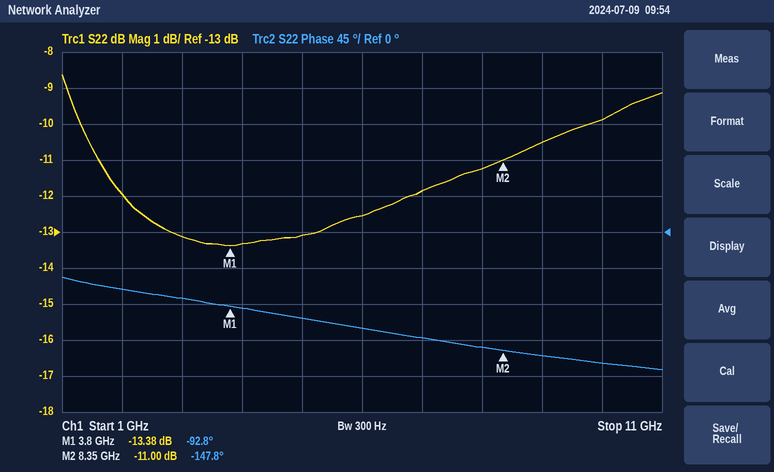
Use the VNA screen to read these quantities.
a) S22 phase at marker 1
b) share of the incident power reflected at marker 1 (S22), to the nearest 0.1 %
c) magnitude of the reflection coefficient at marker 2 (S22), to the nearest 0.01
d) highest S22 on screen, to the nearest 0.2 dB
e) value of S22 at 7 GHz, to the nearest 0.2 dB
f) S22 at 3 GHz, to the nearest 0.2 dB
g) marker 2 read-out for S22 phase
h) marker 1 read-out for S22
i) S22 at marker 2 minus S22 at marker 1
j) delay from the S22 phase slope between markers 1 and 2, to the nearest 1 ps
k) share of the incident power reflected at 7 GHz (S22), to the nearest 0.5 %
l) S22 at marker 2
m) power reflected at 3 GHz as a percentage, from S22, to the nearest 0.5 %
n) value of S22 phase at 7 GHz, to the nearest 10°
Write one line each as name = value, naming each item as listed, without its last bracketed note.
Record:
S22 phase at marker 1 = -92.8°
share of the incident power reflected at marker 1 (S22), to the nearest 0.1 % = 4.6 %
magnitude of the reflection coefficient at marker 2 (S22), to the nearest 0.01 = 0.28
highest S22 on screen, to the nearest 0.2 dB = -8.6 dB
value of S22 at 7 GHz, to the nearest 0.2 dB = -11.8 dB
S22 at 3 GHz, to the nearest 0.2 dB = -13.2 dB
marker 2 read-out for S22 phase = -147.8°
marker 1 read-out for S22 = -13.38 dB
S22 at marker 2 minus S22 at marker 1 = 2.38 dB
delay from the S22 phase slope between markers 1 and 2, to the nearest 1 ps = 34 ps
share of the incident power reflected at 7 GHz (S22), to the nearest 0.5 % = 6.5 %
S22 at marker 2 = -11.00 dB
power reflected at 3 GHz as a percentage, from S22, to the nearest 0.5 % = 5.0 %
value of S22 phase at 7 GHz, to the nearest 10° = -130°
